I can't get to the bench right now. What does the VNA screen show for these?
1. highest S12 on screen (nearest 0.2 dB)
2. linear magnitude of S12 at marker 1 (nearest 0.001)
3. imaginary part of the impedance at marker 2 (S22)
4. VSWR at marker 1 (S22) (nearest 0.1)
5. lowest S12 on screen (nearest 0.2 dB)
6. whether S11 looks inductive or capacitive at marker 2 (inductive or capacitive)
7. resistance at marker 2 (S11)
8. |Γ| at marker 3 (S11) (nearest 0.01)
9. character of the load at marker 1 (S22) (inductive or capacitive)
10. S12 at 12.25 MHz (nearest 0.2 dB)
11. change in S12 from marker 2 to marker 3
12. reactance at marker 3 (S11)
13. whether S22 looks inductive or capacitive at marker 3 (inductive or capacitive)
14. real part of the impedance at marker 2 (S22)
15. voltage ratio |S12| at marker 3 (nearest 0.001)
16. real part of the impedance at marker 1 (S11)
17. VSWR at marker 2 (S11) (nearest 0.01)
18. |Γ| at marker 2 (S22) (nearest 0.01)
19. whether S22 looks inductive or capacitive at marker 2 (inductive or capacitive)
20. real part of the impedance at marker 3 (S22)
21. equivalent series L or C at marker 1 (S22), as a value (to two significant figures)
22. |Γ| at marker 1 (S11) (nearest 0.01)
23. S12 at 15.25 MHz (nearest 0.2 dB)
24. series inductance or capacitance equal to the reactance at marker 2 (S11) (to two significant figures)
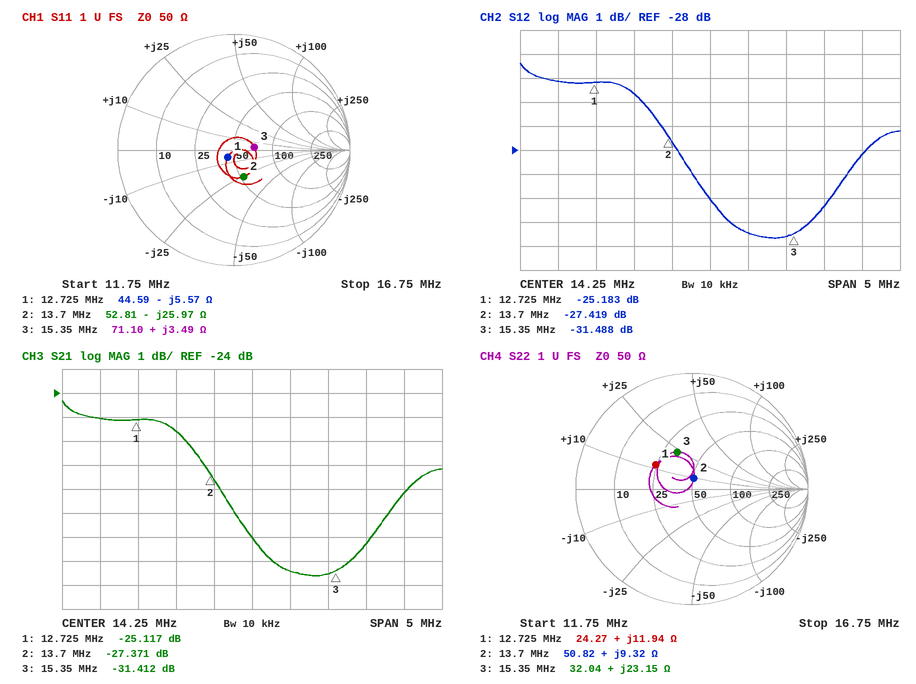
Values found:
-24.4 dB
0.055
+9.32 Ω
2.2
-31.6 dB
capacitive
52.81 Ω
0.18
inductive
-25.2 dB
-4.069 dB
+3.49 Ω
inductive
50.82 Ω
0.027
44.59 Ω
1.65
0.09
inductive
32.04 Ω
150 nH
0.08
-31.6 dB
450 pF
